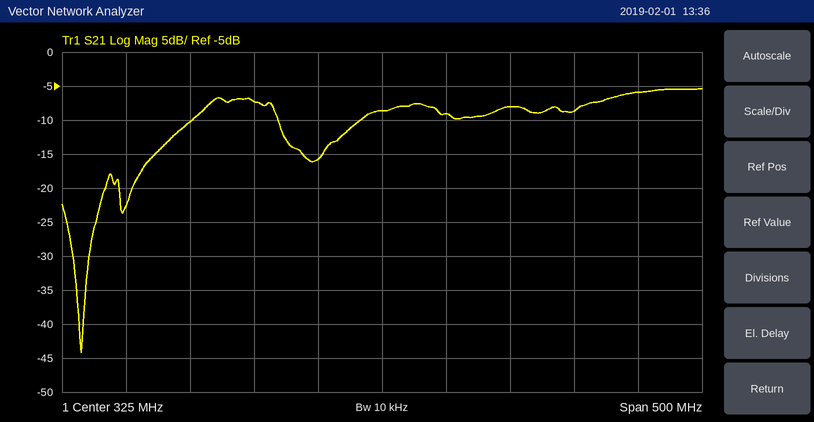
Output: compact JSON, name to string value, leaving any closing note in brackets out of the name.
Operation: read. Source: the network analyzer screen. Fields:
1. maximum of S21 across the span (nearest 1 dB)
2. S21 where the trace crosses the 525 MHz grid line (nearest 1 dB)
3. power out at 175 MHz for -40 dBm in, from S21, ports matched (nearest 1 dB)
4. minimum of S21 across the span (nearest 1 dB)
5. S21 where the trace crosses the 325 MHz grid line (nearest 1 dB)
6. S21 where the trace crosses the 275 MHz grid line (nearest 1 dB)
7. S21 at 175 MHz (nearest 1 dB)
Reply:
{"maximum of S21 across the span": "-5 dB", "S21 where the trace crosses the 525 MHz grid line": "-6 dB", "power out at 175 MHz for -40 dBm in, from S21, ports matched": "-50 dBm", "minimum of S21 across the span": "-44 dB", "S21 where the trace crosses the 325 MHz grid line": "-9 dB", "S21 where the trace crosses the 275 MHz grid line": "-16 dB", "S21 at 175 MHz": "-10 dB"}
